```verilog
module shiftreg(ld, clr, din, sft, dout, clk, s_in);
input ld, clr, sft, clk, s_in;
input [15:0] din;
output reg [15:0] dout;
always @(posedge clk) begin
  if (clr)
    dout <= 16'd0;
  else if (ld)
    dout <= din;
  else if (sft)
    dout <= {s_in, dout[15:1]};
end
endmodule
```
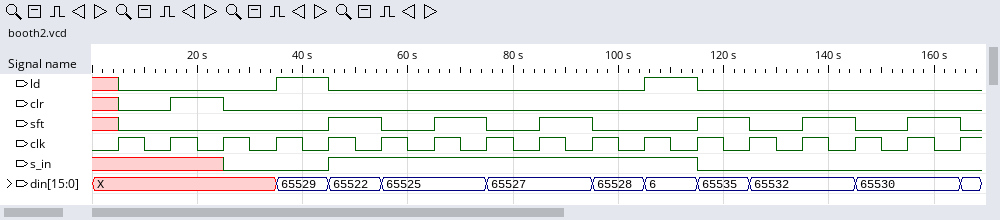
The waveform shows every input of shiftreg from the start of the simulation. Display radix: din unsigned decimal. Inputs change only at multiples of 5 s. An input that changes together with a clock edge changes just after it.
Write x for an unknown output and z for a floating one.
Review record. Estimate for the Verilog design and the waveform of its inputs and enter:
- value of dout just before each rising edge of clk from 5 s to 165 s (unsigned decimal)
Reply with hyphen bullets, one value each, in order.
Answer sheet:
- x, x, x, 0, 0, 65529, 65532, 65532, 65534, 65534, 65535, 65535, 6, 3, 3, 1, 1
